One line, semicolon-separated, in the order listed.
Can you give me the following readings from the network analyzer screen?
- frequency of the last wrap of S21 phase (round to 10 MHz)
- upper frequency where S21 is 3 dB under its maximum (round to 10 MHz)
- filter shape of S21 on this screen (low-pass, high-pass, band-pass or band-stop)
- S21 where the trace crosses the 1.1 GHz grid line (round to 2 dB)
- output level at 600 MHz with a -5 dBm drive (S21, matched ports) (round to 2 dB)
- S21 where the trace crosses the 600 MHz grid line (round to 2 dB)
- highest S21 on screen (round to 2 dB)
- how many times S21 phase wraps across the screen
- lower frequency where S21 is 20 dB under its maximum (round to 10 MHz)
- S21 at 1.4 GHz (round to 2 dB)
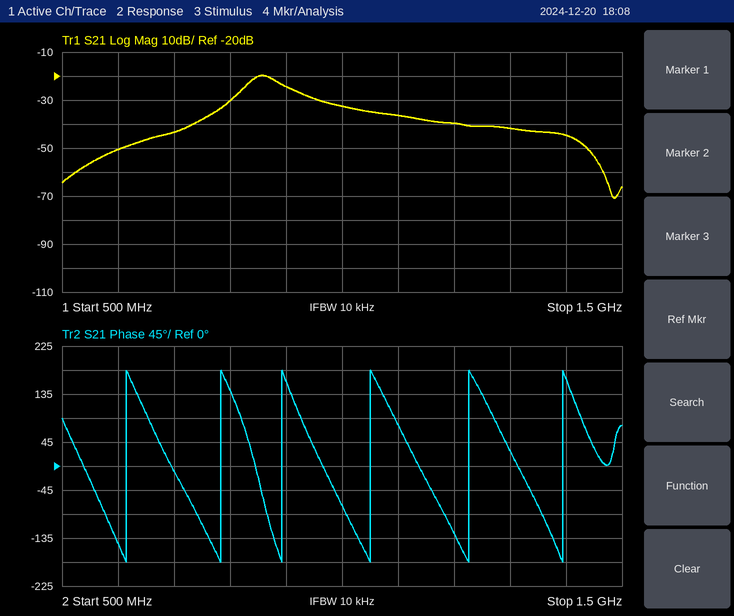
1.39 GHz; 890 MHz; band-pass; -36 dB; -56 dBm; -50 dB; -20 dB; 6; 740 MHz; -44 dB
